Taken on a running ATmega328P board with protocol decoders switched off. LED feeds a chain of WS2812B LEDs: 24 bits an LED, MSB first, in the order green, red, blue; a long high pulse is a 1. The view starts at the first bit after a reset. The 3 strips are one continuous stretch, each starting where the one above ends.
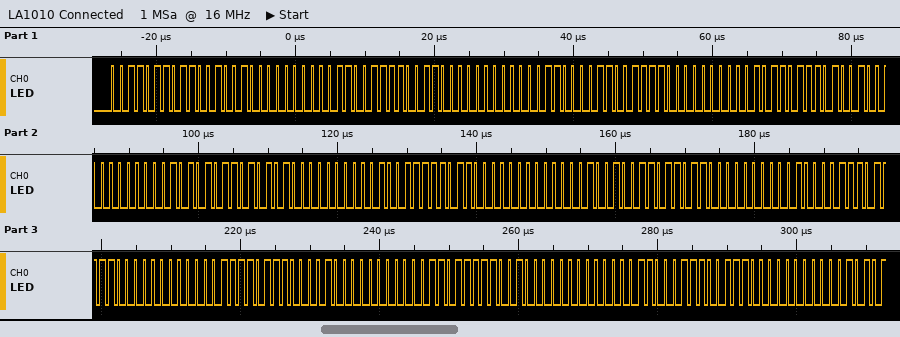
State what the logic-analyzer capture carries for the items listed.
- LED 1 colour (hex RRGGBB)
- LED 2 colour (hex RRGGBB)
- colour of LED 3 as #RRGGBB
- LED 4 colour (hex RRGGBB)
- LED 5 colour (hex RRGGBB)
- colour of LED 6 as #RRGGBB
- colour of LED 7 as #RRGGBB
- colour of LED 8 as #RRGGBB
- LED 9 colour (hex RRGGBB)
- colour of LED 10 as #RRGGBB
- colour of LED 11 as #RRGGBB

#C93600
#CC3300
#CF3000
#D22D00
#D52A00
#D82700
#DB2400
#DE2100
#E11E00
#E41B00
#E71800
